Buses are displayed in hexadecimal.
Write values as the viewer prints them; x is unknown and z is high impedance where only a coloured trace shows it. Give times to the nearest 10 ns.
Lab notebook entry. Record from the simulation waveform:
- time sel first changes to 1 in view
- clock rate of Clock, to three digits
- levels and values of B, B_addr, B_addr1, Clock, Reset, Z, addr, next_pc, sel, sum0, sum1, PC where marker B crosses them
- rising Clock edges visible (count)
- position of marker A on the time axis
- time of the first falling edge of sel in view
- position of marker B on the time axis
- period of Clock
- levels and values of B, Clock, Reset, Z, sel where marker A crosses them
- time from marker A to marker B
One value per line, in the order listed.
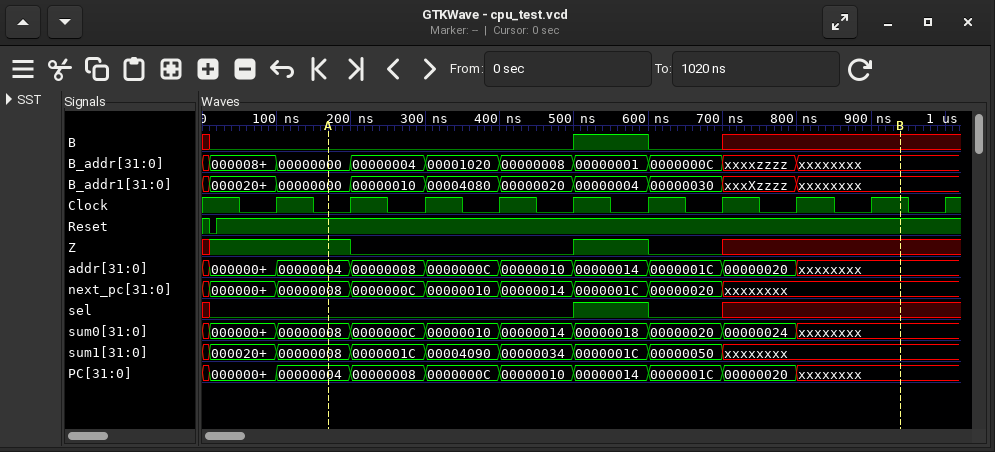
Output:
500 ns
10.0 MHz
B=x, B_addr=xxxxxxxx, B_addr1=xxxxxxxx, Clock=1, Reset=1, Z=x, addr=xxxxxxxx, next_pc=xxxxxxxx, sel=x, sum0=xxxxxxxx, sum1=xxxxxxxx, PC=xxxxxxxx
10
170 ns
600 ns
940 ns
100 ns
B=0, Clock=0, Reset=1, Z=1, sel=0
770 ns
